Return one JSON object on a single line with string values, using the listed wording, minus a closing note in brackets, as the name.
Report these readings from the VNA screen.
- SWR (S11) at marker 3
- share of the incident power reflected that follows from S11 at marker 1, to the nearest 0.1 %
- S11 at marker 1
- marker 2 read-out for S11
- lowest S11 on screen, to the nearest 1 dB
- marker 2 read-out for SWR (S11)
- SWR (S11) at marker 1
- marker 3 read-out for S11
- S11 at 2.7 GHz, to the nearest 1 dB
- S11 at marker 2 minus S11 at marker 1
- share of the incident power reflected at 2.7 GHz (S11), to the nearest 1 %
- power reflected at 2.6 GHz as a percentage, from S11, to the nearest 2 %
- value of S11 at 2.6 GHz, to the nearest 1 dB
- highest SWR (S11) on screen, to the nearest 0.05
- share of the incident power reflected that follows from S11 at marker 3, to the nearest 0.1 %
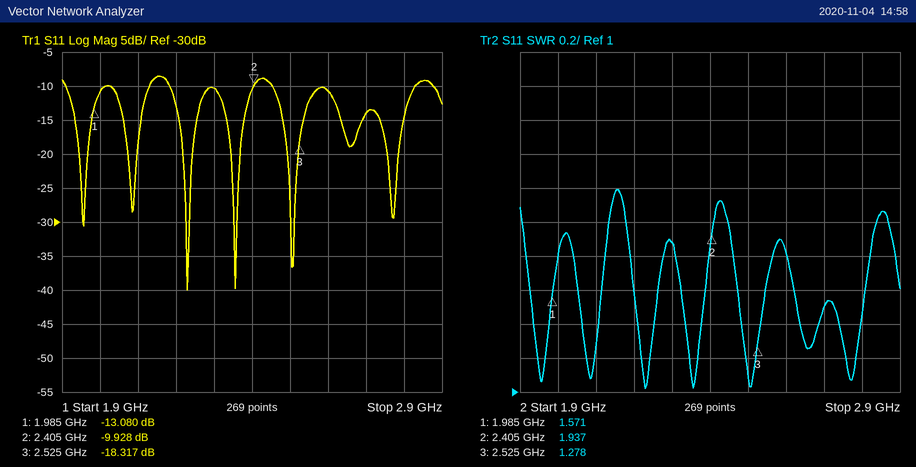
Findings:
{"SWR (S11) at marker 3": "1.278", "share of the incident power reflected that follows from S11 at marker 1, to the nearest 0.1 %": "4.9 %", "S11 at marker 1": "-13.080 dB", "marker 2 read-out for S11": "-9.928 dB", "lowest S11 on screen, to the nearest 1 dB": "-40 dB", "marker 2 read-out for SWR": "1.937", "SWR (S11) at marker 1": "1.571", "marker 3 read-out for S11": "-18.317 dB", "S11 at 2.7 GHz, to the nearest 1 dB": "-14 dB", "S11 at marker 2 minus S11 at marker 1": "3.152 dB", "share of the incident power reflected at 2.7 GHz (S11), to the nearest 1 %": "4 %", "power reflected at 2.6 GHz as a percentage, from S11, to the nearest 2 %": "8 %", "value of S11 at 2.6 GHz, to the nearest 1 dB": "-11 dB", "highest SWR (S11) on screen, to the nearest 0.05": "2.20", "share of the incident power reflected that follows from S11 at marker 3, to the nearest 0.1 %": "1.5 %"}
